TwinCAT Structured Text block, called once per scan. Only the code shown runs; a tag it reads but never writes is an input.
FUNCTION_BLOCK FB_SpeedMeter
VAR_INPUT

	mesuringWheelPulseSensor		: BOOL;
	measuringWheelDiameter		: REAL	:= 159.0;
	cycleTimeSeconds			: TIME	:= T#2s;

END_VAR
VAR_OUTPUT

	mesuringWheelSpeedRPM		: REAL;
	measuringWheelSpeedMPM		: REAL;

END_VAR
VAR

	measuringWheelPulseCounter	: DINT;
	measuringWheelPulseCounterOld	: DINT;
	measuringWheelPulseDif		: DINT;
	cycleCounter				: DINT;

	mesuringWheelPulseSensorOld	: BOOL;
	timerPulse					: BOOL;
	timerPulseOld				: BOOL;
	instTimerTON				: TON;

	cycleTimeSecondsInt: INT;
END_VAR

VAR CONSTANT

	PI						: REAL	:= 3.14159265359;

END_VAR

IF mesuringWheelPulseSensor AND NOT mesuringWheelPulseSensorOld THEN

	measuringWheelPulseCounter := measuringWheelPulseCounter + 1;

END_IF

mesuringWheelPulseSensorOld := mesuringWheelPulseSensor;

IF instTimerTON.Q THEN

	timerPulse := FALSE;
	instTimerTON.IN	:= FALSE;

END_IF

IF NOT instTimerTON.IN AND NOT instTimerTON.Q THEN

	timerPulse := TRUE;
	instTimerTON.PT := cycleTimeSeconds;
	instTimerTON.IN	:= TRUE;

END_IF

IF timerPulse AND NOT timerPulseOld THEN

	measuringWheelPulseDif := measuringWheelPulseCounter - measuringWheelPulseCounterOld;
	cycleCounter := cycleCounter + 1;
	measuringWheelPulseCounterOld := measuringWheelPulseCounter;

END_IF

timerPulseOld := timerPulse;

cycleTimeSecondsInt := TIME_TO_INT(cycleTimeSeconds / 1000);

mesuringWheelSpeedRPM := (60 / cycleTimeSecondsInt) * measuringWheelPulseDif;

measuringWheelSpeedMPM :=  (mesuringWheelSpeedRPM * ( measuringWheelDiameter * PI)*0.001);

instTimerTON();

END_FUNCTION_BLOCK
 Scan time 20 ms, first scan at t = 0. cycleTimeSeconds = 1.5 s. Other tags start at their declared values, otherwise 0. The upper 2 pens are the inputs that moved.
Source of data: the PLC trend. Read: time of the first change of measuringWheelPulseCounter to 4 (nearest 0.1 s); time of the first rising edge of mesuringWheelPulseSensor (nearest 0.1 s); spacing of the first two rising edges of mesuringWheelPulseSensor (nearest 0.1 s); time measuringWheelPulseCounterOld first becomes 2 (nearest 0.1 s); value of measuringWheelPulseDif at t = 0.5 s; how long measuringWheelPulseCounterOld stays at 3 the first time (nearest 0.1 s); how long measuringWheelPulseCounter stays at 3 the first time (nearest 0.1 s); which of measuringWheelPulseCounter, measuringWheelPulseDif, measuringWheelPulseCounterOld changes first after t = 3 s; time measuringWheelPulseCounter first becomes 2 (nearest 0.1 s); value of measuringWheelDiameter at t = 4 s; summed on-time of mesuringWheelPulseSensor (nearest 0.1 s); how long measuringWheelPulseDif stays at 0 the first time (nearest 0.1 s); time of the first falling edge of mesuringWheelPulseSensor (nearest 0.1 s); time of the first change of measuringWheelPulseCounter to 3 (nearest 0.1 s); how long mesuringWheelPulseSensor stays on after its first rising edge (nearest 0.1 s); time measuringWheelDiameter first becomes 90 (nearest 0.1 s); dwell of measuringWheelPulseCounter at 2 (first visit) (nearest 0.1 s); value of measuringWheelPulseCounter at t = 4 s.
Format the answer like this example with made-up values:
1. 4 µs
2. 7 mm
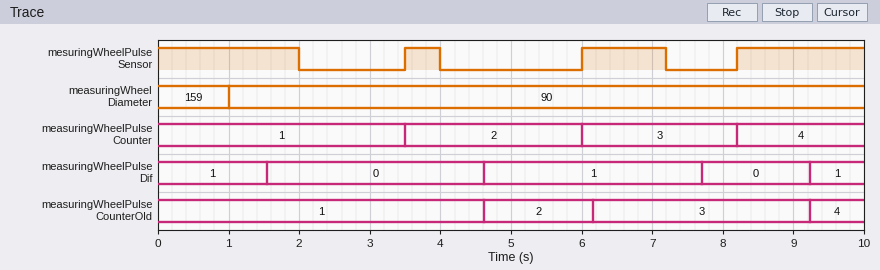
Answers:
1. 8.2 s
2. 3.5 s
3. 2.5 s
4. 4.6 s
5. 1
6. 3.1 s
7. 2.2 s
8. measuringWheelPulseCounter
9. 3.5 s
10. 90
11. 5.5 s
12. 3.1 s
13. 2.0 s
14. 6.0 s
15. 0.5 s
16. 1.0 s
17. 2.5 s
18. 2
